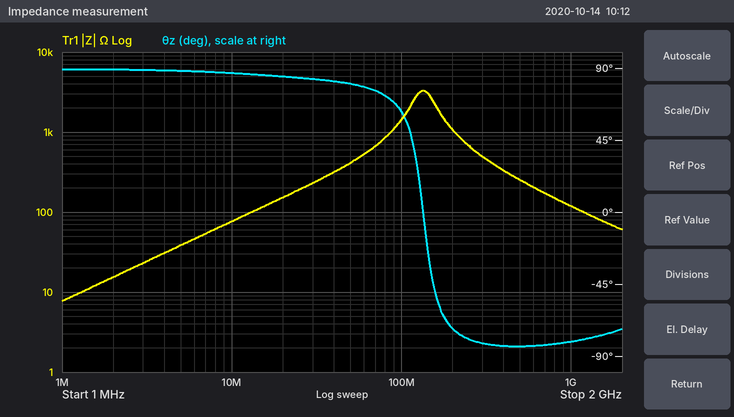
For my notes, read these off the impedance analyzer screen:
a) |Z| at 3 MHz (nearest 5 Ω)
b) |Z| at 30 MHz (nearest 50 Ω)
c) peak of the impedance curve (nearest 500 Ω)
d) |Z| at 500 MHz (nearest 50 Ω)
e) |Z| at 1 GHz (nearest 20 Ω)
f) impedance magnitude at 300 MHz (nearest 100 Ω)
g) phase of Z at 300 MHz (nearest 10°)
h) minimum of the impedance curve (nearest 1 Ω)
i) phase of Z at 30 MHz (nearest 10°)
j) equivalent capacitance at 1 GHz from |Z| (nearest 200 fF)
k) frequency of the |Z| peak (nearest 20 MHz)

25 Ω
250 Ω
3.5 kΩ
250 Ω
120 Ω
500 Ω
-80°
8 Ω
80°
1.4 pF
140 MHz
